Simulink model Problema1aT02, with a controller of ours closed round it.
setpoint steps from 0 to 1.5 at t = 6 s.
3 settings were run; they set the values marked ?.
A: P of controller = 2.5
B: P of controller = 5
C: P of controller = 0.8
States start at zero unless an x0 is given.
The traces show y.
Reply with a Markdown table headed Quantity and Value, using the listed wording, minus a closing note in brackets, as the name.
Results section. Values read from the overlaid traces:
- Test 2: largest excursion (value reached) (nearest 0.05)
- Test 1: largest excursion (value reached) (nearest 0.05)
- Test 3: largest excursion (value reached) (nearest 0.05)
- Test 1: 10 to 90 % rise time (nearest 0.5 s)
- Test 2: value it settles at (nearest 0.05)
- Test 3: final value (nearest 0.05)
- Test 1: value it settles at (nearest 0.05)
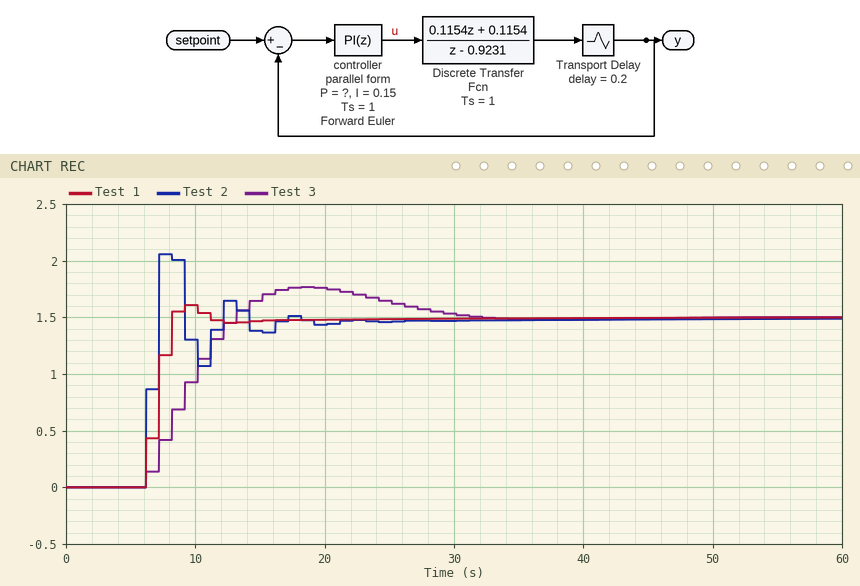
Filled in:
| Quantity | Value |
|---|---|
| Test 2: largest excursion (value reached) | 2.05 |
| Test 1: largest excursion (value reached) | 1.60 |
| Test 3: largest excursion (value reached) | 1.75 |
| Test 1: 10 to 90 % rise time | 2.0 s |
| Test 2: value it settles at | 1.50 |
| Test 3: final value | 1.50 |
| Test 1: value it settles at | 1.50 |
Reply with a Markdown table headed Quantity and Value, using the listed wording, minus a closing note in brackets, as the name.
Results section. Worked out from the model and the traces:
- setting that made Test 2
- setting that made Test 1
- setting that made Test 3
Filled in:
| Quantity | Value |
|---|---|
| setting that made Test 2 | B |
| setting that made Test 1 | A |
| setting that made Test 3 | C |
